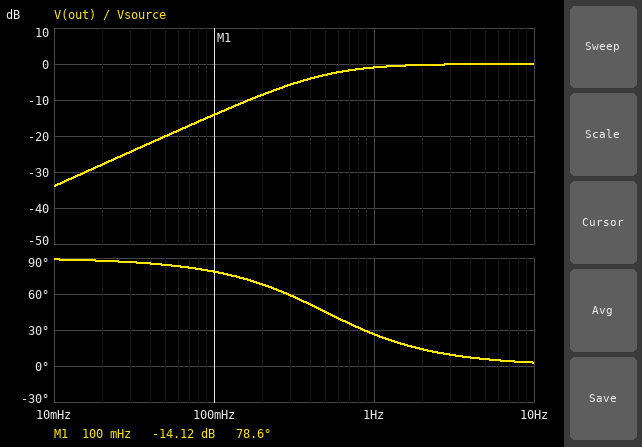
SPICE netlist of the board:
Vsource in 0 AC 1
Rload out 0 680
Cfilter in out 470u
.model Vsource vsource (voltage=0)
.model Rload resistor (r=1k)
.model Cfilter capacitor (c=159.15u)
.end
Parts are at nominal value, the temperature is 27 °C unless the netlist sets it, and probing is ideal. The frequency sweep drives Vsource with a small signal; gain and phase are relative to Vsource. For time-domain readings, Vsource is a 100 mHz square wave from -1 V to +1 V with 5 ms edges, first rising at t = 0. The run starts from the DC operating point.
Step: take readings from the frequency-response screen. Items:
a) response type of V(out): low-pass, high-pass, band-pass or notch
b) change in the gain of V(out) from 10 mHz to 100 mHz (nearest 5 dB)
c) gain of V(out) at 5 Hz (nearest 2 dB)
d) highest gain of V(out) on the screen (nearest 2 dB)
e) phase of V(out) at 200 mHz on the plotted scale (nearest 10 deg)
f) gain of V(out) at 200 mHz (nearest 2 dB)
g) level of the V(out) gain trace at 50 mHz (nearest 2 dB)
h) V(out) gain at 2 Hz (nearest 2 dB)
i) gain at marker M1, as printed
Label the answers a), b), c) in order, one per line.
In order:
a) high-pass
b) 20 dB
c) 0 dB
d) 0 dB
e) 70 deg
f) -8 dB
g) -20 dB
h) 0 dB
i) -14.12 dB
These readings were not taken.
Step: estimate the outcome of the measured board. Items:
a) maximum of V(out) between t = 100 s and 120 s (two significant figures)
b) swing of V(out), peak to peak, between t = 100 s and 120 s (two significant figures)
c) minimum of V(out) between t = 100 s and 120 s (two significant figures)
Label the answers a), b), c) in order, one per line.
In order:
a) 2.0 V
b) 4.0 V
c) -2.0 V
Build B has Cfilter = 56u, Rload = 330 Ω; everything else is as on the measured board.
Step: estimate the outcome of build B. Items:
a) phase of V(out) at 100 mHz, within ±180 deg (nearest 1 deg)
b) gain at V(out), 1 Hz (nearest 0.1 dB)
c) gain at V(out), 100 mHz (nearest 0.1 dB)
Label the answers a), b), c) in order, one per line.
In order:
a) 89 deg
b) -18.8 dB
c) -38.7 dB
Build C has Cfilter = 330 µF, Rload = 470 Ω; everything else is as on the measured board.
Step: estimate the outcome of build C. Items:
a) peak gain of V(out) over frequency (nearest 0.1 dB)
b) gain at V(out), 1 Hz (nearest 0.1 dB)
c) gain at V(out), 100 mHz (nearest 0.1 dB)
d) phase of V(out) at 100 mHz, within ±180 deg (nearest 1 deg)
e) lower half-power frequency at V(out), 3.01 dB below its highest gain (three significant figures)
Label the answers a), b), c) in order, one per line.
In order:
a) 0 dB
b) -3.1 dB
c) -20.3 dB
d) 84 deg
e) 1.03 Hz
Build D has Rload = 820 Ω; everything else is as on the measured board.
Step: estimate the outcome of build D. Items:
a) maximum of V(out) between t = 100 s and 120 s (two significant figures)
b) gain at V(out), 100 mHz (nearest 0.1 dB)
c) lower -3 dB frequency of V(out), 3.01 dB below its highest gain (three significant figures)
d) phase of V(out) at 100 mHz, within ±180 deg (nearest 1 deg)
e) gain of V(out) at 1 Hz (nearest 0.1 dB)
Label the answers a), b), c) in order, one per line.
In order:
a) 2.0 V
b) -12.6 dB
c) 413 mHz
d) 76 deg
e) -0.7 dB
